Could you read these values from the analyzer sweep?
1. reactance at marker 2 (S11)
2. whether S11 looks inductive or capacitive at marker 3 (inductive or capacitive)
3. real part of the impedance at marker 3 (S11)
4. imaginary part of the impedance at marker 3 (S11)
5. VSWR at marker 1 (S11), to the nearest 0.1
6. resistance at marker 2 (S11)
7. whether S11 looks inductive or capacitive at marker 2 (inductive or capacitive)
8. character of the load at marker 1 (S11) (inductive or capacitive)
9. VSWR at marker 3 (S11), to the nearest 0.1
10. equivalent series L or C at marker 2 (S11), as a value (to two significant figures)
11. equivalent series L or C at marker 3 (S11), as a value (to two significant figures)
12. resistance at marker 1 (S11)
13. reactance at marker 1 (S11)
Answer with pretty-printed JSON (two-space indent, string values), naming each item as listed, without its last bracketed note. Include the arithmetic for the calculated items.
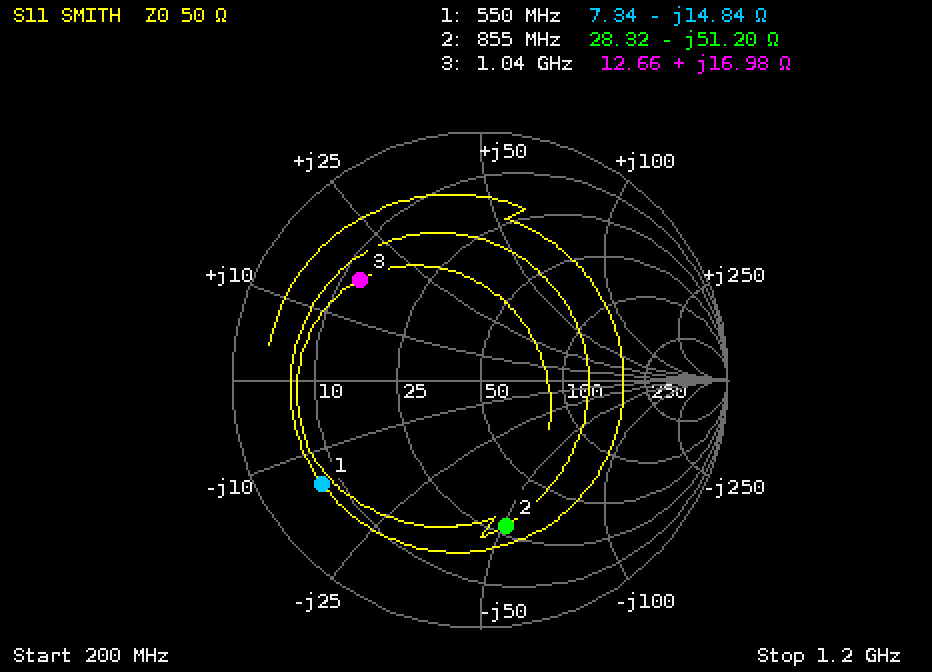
{
  "reactance at marker 2": "-51.20 Ω",
  "whether S11 looks inductive or capacitive at marker 3": "inductive",
  "real part of the impedance at marker 3": "12.66 Ω",
  "imaginary part of the impedance at marker 3": "+16.98 Ω",
  "VSWR at marker 1 (S11), to the nearest 0.1": "7.4",
  "resistance at marker 2": "28.32 Ω",
  "whether S11 looks inductive or capacitive at marker 2": "capacitive",
  "character of the load at marker 1 (S11)": "capacitive",
  "VSWR at marker 3 (S11), to the nearest 0.1": "4.4",
  "equivalent series L or C at marker 2 (S11), as a value": "C = 1/(2π × 855 MHz × 51.2 Ω) ≈ 3.6 pF",
  "equivalent series L or C at marker 3 (S11), as a value": "L = 16.98 Ω/(2π × 1.04 GHz) ≈ 2.6 nH",
  "resistance at marker 1": "7.34 Ω",
  "reactance at marker 1": "-14.84 Ω"
}
